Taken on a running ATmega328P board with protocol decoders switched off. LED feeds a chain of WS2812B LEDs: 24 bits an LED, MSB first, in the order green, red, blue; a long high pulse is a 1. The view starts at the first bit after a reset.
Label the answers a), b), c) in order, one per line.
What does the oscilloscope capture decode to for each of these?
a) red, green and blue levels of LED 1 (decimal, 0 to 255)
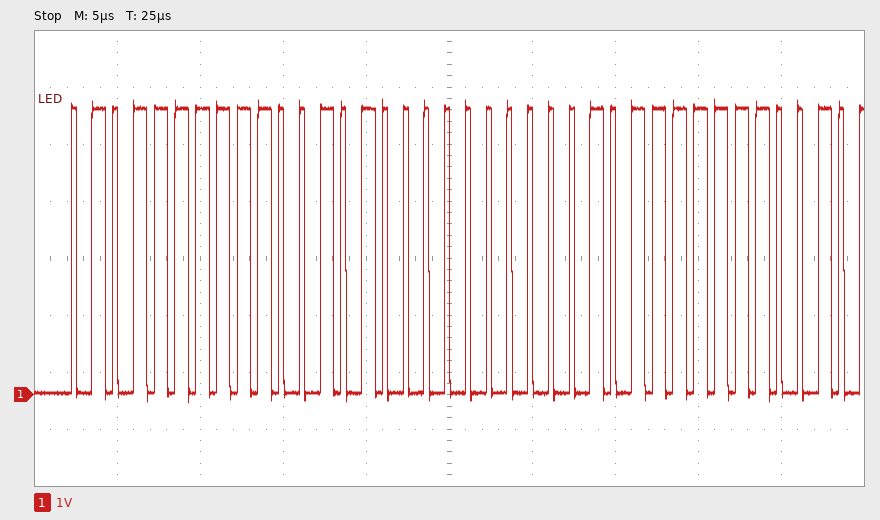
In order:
a) 202, 95, 0
